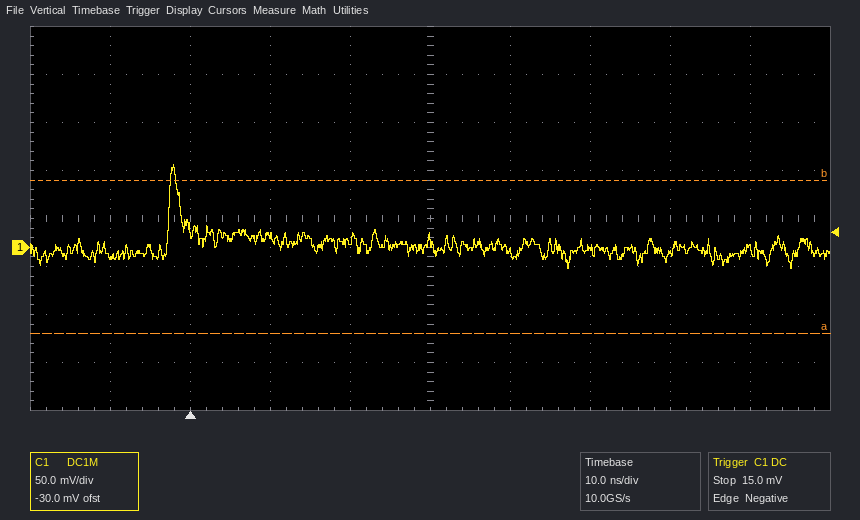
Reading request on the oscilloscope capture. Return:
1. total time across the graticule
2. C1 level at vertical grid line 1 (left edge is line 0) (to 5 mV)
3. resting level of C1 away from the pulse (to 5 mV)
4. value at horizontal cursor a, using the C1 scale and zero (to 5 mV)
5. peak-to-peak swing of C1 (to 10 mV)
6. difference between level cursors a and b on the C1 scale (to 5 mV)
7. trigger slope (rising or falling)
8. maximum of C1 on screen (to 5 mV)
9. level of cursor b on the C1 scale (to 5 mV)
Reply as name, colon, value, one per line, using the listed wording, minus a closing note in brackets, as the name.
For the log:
total time across the graticule: 100 ns
C1 level at vertical grid line 1 (left edge is line 0): -10 mV
resting level of C1 away from the pulse: 0 mV
value at horizontal cursor a, using the C1 scale and zero: -90 mV
peak-to-peak swing of C1: 110 mV
difference between level cursors a and b on the C1 scale: 160 mV
trigger slope: falling
maximum of C1 on screen: 85 mV
level of cursor b on the C1 scale: 70 mV
